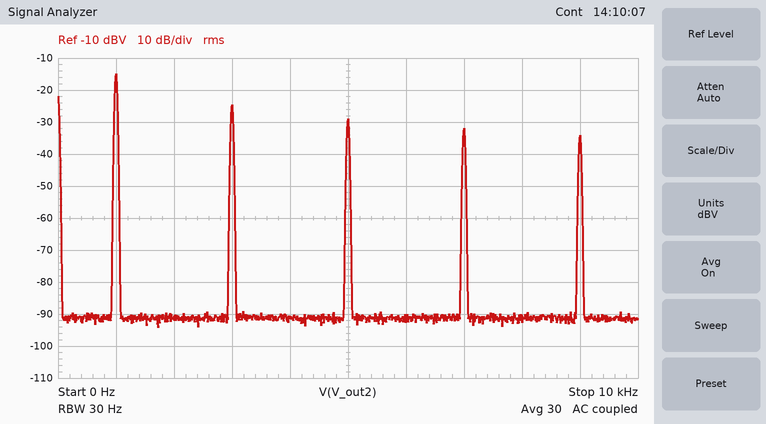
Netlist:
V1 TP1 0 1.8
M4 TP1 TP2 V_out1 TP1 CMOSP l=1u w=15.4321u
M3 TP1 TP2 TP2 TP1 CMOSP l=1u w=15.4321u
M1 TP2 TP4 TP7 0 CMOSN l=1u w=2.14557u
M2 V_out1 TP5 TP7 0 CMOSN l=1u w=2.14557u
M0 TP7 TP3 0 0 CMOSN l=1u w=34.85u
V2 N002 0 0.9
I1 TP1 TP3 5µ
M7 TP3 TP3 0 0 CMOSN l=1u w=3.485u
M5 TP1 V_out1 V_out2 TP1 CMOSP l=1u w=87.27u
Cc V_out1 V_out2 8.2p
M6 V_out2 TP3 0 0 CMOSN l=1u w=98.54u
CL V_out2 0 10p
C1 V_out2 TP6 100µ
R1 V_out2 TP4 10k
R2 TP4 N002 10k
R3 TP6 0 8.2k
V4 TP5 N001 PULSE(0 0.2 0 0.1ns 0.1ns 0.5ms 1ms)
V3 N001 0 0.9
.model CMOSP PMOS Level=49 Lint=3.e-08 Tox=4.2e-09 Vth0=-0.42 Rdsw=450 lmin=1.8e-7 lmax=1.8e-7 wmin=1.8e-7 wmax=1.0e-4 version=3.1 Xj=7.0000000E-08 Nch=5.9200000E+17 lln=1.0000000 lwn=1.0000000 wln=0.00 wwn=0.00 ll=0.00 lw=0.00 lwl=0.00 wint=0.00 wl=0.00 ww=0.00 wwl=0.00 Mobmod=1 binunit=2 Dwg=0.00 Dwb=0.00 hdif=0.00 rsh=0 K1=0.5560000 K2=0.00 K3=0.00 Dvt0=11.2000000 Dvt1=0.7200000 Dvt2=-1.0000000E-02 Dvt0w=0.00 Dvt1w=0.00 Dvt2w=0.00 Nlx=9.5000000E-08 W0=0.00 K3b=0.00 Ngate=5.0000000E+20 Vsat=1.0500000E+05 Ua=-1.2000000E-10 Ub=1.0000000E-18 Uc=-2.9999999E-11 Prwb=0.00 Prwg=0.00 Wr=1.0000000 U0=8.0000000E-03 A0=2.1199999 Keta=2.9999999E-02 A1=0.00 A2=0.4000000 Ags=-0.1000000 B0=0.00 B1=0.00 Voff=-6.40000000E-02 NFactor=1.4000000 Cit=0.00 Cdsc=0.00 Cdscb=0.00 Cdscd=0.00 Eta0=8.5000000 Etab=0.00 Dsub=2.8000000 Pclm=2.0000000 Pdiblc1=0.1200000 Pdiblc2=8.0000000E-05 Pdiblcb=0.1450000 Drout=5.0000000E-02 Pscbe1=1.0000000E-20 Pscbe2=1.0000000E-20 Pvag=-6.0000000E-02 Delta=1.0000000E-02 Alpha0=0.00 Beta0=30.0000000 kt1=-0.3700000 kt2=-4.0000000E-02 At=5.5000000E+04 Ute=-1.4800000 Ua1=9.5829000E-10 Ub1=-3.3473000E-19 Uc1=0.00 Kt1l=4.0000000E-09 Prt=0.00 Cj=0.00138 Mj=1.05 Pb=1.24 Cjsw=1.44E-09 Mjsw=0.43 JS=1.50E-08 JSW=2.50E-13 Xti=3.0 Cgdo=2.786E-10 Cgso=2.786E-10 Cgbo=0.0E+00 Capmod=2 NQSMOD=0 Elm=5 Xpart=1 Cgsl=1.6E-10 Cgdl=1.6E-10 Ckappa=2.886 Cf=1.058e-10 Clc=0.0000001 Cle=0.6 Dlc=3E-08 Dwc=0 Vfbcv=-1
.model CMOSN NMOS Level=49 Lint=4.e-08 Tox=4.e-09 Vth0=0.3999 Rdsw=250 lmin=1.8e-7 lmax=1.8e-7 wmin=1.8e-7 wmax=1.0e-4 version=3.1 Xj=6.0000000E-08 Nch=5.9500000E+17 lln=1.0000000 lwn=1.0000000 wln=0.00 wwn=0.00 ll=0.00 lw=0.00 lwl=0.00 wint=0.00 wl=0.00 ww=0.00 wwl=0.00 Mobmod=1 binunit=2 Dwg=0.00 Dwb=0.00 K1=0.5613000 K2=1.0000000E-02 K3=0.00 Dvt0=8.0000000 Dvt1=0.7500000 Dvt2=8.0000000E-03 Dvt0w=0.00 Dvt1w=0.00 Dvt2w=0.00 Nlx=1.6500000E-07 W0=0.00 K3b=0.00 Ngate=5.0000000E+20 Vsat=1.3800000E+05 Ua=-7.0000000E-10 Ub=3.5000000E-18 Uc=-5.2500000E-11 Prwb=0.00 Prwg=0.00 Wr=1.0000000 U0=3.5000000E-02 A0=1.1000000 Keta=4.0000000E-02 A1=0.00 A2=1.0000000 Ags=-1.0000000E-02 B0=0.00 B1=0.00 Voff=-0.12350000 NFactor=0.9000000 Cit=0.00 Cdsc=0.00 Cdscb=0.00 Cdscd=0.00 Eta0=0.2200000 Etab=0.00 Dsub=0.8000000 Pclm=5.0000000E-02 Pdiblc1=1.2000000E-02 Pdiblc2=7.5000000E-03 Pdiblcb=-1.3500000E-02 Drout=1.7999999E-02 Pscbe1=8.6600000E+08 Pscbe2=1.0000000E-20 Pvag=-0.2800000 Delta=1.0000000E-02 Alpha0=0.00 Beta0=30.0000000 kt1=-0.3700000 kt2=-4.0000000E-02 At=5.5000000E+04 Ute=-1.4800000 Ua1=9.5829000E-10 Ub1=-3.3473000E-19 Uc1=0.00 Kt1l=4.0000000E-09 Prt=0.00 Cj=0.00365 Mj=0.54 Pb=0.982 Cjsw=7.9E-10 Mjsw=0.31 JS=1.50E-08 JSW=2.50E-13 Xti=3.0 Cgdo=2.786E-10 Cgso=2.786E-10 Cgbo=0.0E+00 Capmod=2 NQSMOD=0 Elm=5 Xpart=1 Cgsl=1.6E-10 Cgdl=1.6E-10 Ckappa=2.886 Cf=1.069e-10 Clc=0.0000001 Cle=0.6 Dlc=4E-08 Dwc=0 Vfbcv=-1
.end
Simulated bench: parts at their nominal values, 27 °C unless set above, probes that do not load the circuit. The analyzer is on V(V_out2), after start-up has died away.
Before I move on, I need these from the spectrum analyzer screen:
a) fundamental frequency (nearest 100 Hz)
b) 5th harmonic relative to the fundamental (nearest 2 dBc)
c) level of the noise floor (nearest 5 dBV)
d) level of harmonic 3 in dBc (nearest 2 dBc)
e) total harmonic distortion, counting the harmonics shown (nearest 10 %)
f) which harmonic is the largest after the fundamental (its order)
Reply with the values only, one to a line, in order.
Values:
1.0 kHz
-14 dBc
-90 dBV
-10 dBc
40 %
3
